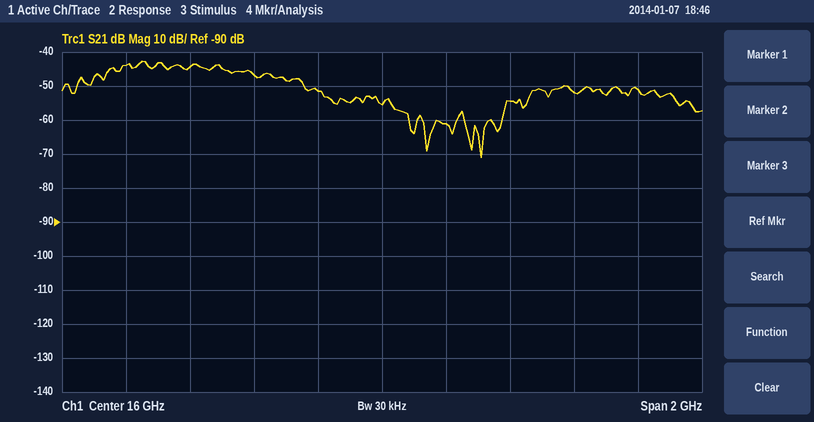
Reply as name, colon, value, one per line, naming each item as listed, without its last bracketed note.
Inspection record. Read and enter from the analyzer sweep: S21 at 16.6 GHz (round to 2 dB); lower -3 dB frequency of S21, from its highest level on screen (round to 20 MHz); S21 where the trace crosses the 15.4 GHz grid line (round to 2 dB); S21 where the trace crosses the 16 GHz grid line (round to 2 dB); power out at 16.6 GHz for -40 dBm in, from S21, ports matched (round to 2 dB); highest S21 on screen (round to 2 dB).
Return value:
S21 at 16.6 GHz: -52 dB
lower -3 dB frequency of S21, from its highest level on screen: 15.14 GHz
S21 where the trace crosses the 15.4 GHz grid line: -44 dB
S21 where the trace crosses the 16 GHz grid line: -56 dB
power out at 16.6 GHz for -40 dBm in, from S21, ports matched: -92 dBm
highest S21 on screen: -42 dB
